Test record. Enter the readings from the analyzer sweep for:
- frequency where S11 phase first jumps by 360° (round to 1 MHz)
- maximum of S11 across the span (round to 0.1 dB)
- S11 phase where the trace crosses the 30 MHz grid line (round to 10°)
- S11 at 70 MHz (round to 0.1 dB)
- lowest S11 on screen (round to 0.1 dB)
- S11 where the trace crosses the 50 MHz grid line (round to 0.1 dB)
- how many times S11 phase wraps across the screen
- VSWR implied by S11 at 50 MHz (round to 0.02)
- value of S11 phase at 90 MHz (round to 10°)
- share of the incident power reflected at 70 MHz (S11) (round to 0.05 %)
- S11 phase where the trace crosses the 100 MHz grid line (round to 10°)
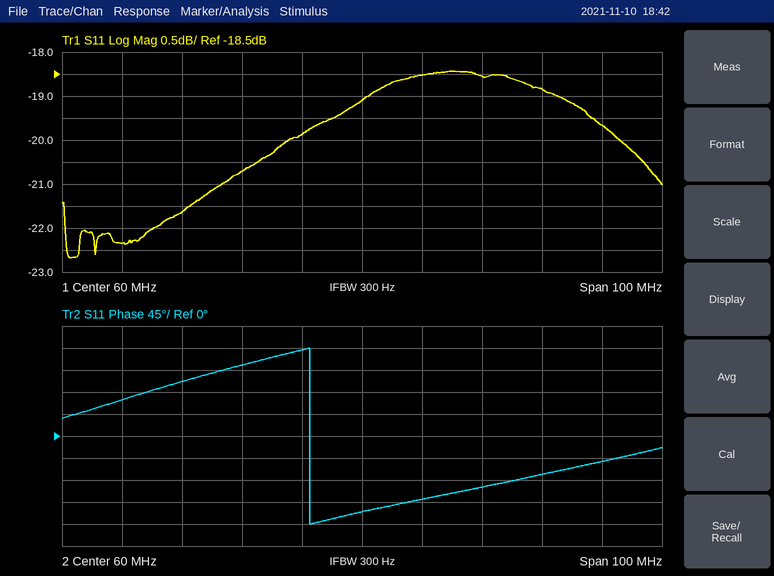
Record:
51 MHz
-18.4 dB
110°
-18.5 dB
-22.7 dB
-19.9 dB
1
1.22
-80°
1.40 %
-50°
